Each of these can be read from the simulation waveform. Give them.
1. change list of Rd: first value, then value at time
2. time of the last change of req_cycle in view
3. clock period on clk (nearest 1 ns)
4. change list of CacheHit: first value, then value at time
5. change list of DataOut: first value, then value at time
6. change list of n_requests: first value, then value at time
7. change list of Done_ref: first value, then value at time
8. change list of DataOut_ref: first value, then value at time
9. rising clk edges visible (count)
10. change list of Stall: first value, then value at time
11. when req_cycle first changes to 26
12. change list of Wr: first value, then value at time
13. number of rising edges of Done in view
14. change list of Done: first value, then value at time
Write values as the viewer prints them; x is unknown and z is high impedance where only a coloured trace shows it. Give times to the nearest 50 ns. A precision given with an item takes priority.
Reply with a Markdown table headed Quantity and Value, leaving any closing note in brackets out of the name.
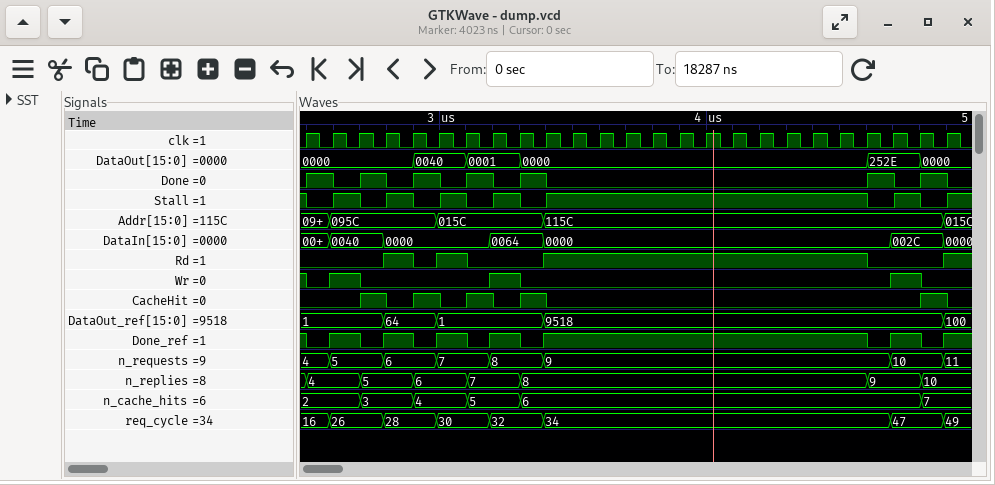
| Quantity | Value |
|---|---|
| change list of Rd: first value, then value at time | 0, 1 at 2800 ns, 0 at 2900 ns, 1 at 3000 ns, 0 at 3100 ns, 1 at 3400 ns, 0 at 4600 ns, 1 at 4900 ns |
| time of the last change of req_cycle in view | 4900 ns |
| clock period on clk | 100 ns |
| change list of CacheHit: first value, then value at time | 0, 1 at 2700 ns, 0 at 2800 ns, 1 at 2900 ns, 0 at 3000 ns, 1 at 3100 ns, 0 at 3200 ns, 1 at 3300 ns, 0 at 3400 ns, 1 at 4800 ns, 0 at 4900 ns |
| change list of DataOut: first value, then value at time | 0000, 0040 at 2900 ns, 0001 at 3100 ns, 0000 at 3300 ns, 252E at 4600 ns, 0000 at 4800 ns |
| change list of n_requests: first value, then value at time | 4, 5 at 2600 ns, 6 at 2800 ns, 7 at 3000 ns, 8 at 3200 ns, 9 at 3400 ns, 10 at 4700 ns, 11 at 4900 ns |
| change list of Done_ref: first value, then value at time | 1, 0 at 2500 ns, 1 at 2600 ns, 0 at 2700 ns, 1 at 2800 ns, 0 at 2900 ns, 1 at 3000 ns, 0 at 3100 ns, 1 at 3200 ns, 0 at 3300 ns, 1 at 3400 ns, 0 at 4600 ns, 1 at 4700 ns, 0 at 4800 ns, 1 at 4900 ns |
| change list of DataOut_ref: first value, then value at time | 1, 64 at 2800 ns, 1 at 3000 ns, 9518 at 3400 ns, 100 at 4900 ns |
| rising clk edges visible | 25 |
| change list of Stall: first value, then value at time | 1, 0 at 2500 ns, 1 at 2600 ns, 0 at 2700 ns, 1 at 2800 ns, 0 at 2900 ns, 1 at 3000 ns, 0 at 3100 ns, 1 at 3200 ns, 0 at 3300 ns, 1 at 3400 ns, 0 at 4600 ns, 1 at 4700 ns, 0 at 4800 ns, 1 at 4900 ns |
| when req_cycle first changes to 26 | 2600 ns |
| change list of Wr: first value, then value at time | 1, 0 at 2500 ns, 1 at 2600 ns, 0 at 2700 ns, 1 at 3200 ns, 0 at 3300 ns, 1 at 4700 ns, 0 at 4800 ns |
| number of rising edges of Done in view | 7 |
| change list of Done: first value, then value at time | 0, 1 at 2500 ns, 0 at 2600 ns, 1 at 2700 ns, 0 at 2800 ns, 1 at 2900 ns, 0 at 3000 ns, 1 at 3100 ns, 0 at 3200 ns, 1 at 3300 ns, 0 at 3400 ns, 1 at 4600 ns, 0 at 4700 ns, 1 at 4800 ns, 0 at 4900 ns |
